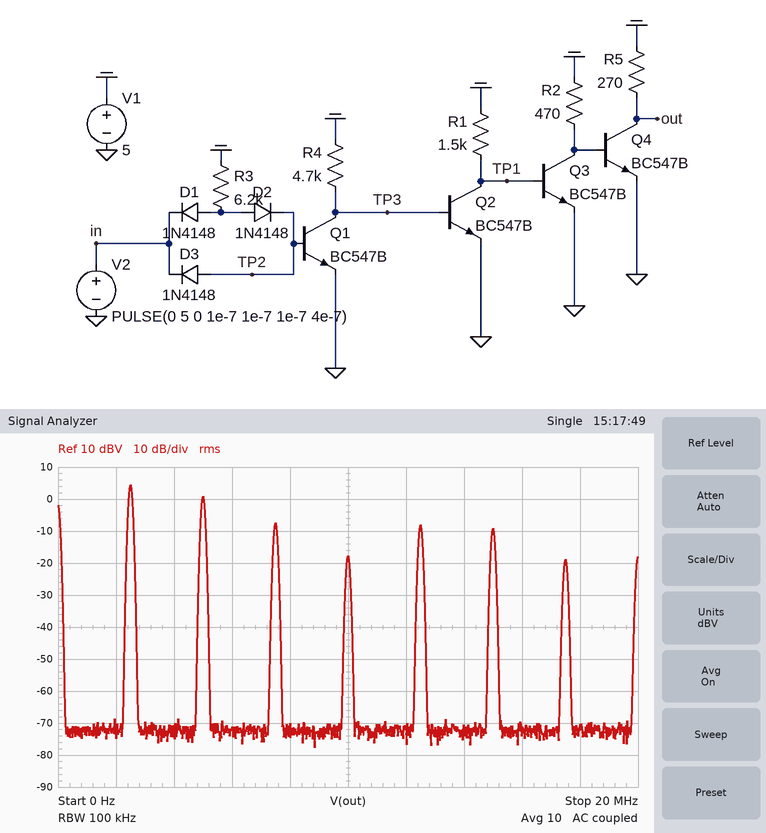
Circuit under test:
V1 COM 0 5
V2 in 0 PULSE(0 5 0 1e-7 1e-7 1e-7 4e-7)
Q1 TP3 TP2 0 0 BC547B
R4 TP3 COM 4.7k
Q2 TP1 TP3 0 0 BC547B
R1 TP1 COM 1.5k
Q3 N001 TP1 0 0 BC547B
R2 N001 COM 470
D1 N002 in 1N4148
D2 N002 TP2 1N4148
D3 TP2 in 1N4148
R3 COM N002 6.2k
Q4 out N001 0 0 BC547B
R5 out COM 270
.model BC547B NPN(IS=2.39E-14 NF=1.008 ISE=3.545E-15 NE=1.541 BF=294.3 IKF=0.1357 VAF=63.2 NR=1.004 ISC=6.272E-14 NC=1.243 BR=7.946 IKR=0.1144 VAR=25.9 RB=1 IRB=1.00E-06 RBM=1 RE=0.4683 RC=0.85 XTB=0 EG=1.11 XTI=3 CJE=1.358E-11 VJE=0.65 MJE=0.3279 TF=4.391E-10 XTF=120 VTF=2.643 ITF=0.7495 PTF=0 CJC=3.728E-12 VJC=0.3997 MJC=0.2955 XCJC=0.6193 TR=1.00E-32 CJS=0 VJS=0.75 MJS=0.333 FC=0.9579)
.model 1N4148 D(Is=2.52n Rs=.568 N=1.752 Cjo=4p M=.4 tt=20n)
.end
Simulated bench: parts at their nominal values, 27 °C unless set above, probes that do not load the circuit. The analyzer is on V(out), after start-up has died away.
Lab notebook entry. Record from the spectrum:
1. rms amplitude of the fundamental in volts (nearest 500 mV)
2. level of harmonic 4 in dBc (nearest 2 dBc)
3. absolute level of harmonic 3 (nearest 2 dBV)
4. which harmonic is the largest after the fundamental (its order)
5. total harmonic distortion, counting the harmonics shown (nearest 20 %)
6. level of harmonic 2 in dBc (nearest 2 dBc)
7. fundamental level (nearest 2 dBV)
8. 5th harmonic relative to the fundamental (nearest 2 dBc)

1.5 V
-22 dBc
-8 dBV
2
80 %
-4 dBc
4 dBV
-12 dBc
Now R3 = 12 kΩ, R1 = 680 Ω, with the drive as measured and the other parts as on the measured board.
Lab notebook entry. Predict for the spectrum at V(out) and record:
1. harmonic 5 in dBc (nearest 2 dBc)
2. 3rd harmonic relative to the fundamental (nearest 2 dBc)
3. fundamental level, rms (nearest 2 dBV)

-14 dBc
-10 dBc
4 dBV
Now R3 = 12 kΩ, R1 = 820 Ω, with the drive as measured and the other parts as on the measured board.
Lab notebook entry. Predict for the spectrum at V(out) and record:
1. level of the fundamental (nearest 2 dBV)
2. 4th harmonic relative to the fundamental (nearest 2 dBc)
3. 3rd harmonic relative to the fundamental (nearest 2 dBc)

4 dBV
-34 dBc
-10 dBc
